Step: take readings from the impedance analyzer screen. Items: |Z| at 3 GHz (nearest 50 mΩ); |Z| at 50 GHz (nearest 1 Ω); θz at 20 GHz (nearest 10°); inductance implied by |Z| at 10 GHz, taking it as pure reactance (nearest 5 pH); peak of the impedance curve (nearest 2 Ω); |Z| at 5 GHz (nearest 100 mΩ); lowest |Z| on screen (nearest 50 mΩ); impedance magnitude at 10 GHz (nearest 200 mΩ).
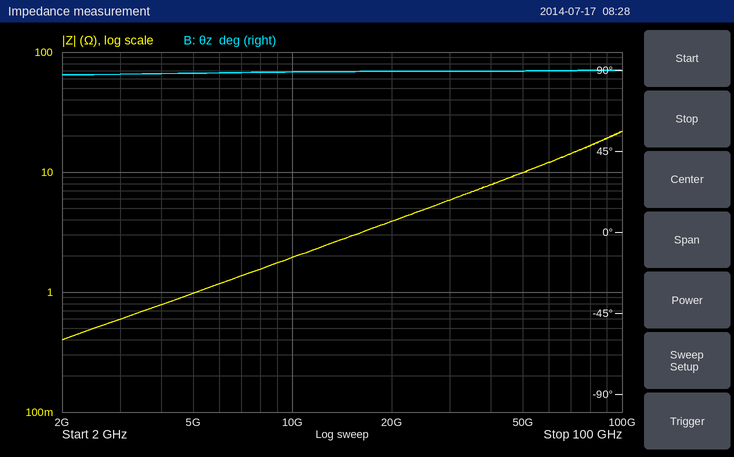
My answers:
600 mΩ
10 Ω
90°
30 pH
22 Ω
1.0 Ω
400 mΩ
2.0 Ω
